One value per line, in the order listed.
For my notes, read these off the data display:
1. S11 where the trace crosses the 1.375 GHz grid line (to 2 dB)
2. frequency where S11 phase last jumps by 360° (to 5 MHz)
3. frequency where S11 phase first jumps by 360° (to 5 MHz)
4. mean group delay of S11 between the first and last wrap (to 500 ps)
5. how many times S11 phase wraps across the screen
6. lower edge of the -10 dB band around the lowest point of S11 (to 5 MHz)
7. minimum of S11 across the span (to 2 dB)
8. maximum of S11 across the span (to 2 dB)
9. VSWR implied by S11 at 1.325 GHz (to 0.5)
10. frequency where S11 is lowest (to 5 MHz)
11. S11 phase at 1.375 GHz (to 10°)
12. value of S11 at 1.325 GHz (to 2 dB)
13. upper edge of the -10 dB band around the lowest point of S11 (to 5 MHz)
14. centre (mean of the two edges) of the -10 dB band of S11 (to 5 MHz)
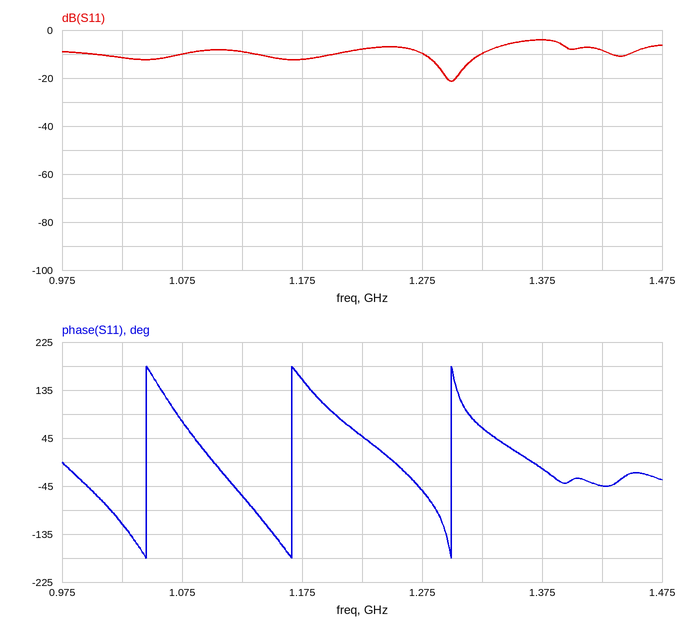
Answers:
-4 dB
1.300 GHz
1.045 GHz
8.0 ns
3
1.275 GHz
-22 dB
-4 dB
2.0
1.300 GHz
-10°
-10 dB
1.325 GHz
1.300 GHz
